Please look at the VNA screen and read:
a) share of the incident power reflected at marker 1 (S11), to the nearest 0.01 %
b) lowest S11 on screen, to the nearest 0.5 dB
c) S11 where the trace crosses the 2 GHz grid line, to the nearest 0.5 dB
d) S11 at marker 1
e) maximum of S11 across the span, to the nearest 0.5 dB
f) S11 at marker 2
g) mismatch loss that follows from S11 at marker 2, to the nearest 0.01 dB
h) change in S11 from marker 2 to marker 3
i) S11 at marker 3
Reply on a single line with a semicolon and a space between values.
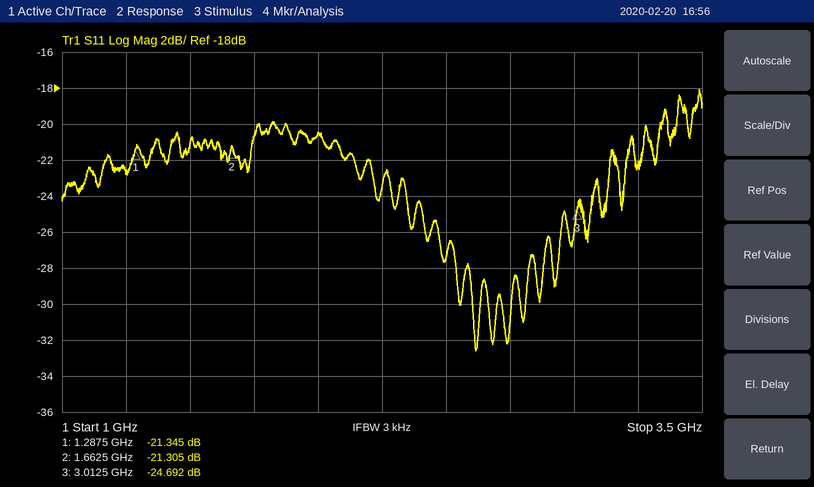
0.73 %; -32.5 dB; -20.5 dB; -21.345 dB; -18.0 dB; -21.305 dB; 0.03 dB; -3.387 dB; -24.692 dB
